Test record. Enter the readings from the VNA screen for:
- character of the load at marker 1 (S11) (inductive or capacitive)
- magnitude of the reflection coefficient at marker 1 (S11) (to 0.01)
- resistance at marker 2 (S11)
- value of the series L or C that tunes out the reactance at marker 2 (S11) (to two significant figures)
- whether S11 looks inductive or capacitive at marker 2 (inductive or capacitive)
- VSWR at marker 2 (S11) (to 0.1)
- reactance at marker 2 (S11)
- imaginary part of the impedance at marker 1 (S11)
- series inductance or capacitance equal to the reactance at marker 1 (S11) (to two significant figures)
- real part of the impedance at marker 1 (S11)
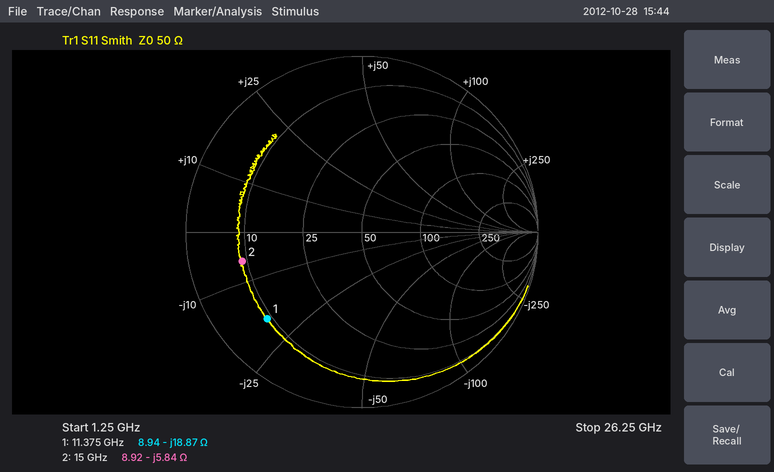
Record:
capacitive
0.73
8.92 Ω
62 pH
capacitive
5.7
-5.84 Ω
-18.87 Ω
740 fF
8.94 Ω
